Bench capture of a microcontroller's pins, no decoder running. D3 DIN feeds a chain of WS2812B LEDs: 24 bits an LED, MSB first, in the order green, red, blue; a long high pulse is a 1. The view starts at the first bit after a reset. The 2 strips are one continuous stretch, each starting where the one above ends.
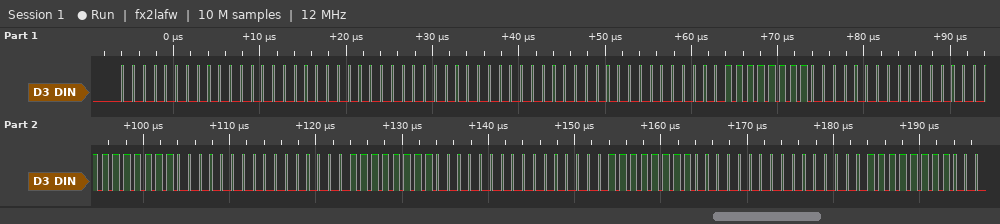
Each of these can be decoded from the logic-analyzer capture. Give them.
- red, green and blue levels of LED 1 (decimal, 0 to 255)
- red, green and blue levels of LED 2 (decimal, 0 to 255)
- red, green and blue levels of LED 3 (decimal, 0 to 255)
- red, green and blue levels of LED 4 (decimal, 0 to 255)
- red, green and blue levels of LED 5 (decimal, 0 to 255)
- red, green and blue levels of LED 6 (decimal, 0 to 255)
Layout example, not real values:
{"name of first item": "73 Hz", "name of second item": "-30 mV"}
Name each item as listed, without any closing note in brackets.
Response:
{"red, green and blue levels of LED 1": "0, 0, 0", "red, green and blue levels of LED 2": "0, 0, 0", "red, green and blue levels of LED 3": "255, 0, 0", "red, green and blue levels of LED 4": "255, 0, 0", "red, green and blue levels of LED 5": "255, 0, 0", "red, green and blue levels of LED 6": "255, 0, 0"}
